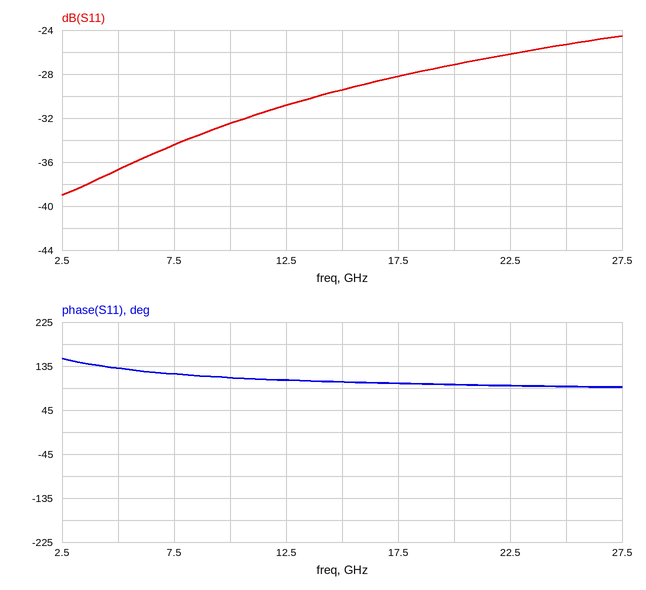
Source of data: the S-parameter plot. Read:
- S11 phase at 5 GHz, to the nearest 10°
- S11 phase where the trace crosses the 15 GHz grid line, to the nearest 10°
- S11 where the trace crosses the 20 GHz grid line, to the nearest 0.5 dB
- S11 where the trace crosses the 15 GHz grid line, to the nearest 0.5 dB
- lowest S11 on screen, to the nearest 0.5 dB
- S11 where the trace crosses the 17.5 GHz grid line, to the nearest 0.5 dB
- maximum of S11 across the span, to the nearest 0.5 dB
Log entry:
130°
100°
-27.0 dB
-29.5 dB
-39.0 dB
-28.0 dB
-24.5 dB
